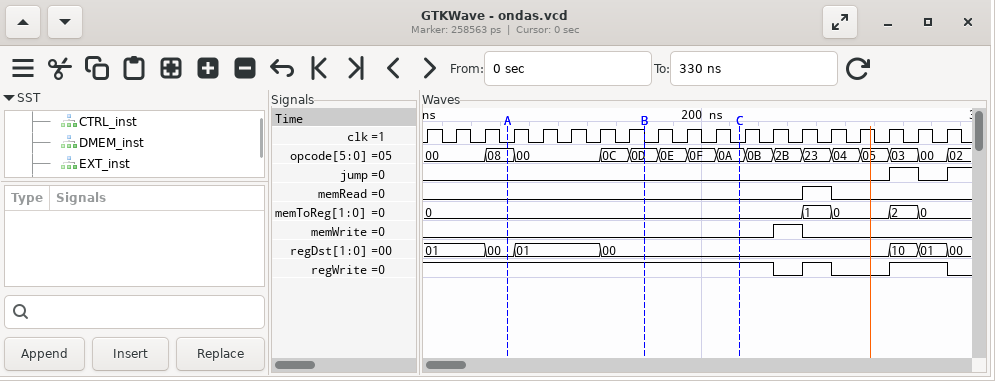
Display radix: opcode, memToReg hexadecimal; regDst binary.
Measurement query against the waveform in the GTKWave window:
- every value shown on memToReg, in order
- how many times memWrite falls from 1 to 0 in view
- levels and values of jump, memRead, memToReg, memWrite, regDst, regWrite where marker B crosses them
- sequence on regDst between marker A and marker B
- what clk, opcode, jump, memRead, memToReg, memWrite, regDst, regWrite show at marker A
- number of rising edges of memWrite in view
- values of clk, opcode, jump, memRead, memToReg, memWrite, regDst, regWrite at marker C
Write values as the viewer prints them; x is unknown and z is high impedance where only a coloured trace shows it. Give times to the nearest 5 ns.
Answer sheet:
0, 1, 0, 2, 0
1
jump=0, memRead=0, memToReg=0, memWrite=0, regDst=00, regWrite=1
00, 01, 00
clk=0, opcode=08, jump=0, memRead=0, memToReg=0, memWrite=0, regDst=00, regWrite=1
1
clk=0, opcode=0A, jump=0, memRead=0, memToReg=0, memWrite=0, regDst=00, regWrite=1
